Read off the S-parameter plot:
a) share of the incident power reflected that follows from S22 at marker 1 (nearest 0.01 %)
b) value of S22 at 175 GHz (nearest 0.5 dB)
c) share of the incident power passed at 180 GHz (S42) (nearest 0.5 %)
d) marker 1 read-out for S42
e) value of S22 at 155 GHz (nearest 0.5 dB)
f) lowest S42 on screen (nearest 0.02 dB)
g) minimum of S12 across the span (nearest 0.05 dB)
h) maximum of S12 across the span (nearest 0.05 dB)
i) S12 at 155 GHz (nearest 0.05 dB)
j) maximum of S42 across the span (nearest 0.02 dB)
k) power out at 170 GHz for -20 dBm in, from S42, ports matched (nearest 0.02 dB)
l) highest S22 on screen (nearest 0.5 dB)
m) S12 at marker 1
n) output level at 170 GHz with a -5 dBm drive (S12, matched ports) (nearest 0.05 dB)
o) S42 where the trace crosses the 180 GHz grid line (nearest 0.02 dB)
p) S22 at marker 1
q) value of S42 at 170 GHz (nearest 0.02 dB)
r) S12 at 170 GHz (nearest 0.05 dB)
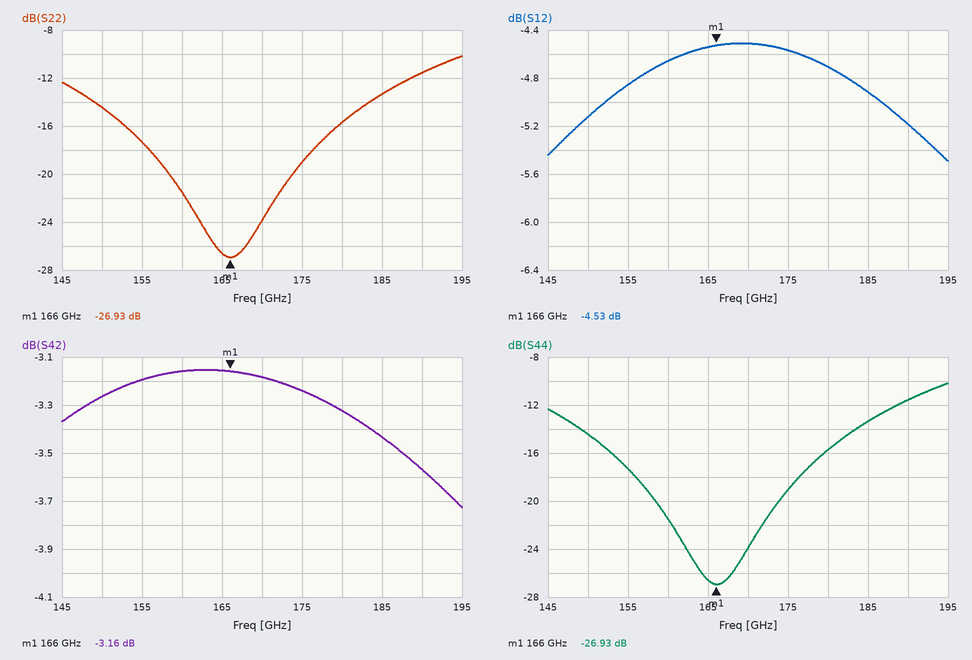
0.20 %
-19.0 dB
46.5 %
-3.16 dB
-17.5 dB
-3.72 dB
-5.50 dB
-4.50 dB
-4.85 dB
-3.16 dB
-23.18 dBm
-10.0 dB
-4.53 dB
-9.50 dBm
-3.32 dB
-26.93 dB
-3.18 dB
-4.50 dB
